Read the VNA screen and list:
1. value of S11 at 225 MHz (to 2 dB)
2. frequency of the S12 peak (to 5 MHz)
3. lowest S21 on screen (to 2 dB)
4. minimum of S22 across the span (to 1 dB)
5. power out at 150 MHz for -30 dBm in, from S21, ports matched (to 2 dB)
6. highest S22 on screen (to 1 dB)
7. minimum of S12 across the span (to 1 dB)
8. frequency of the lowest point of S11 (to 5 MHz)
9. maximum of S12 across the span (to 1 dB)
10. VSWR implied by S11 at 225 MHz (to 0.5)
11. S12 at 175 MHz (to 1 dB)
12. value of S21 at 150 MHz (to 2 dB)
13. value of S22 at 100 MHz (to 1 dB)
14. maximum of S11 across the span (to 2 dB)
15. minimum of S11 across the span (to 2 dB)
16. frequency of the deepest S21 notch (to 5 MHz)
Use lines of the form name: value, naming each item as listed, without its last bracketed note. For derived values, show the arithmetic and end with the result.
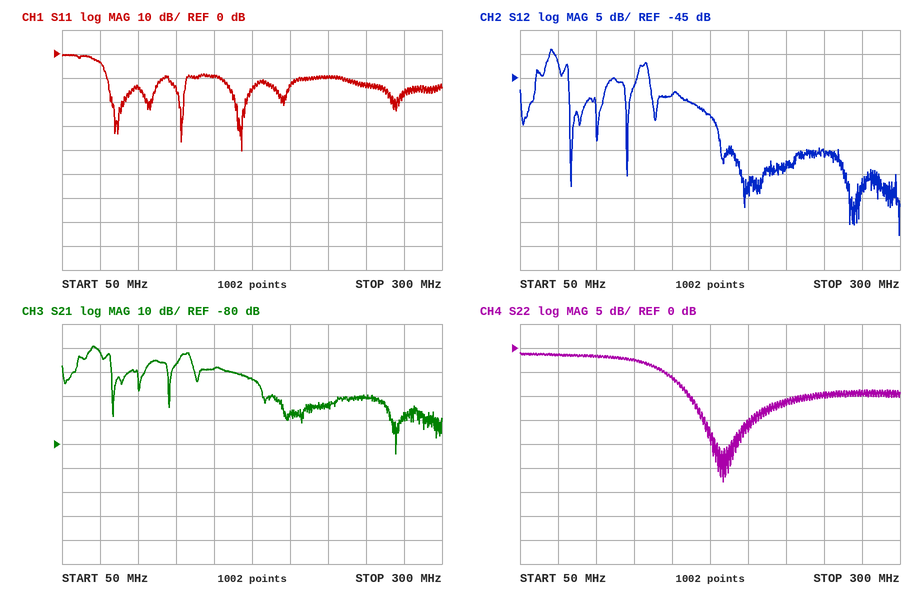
value of S11 at 225 MHz: -10 dB
frequency of the S12 peak: 70 MHz
lowest S21 on screen: -84 dB
minimum of S22 across the span: -28 dB
power out at 150 MHz for -30 dBm in, from S21, ports matched: -30 dBm + (-48 dB) = -78 dBm
highest S22 on screen: -1 dB
minimum of S12 across the span: -78 dB
frequency of the lowest point of S11: 170 MHz
maximum of S12 across the span: -39 dB
VSWR implied by S11 at 225 MHz: |Γ| = 10^(-10/20) = 0.3162; VSWR = (1 + 0.3162)/(1 − 0.3162) ≈ 1.92, so 2.0 to the nearest 0.5
S12 at 175 MHz: -53 dB
value of S21 at 150 MHz: -48 dB
value of S22 at 100 MHz: -2 dB
maximum of S11 across the span: 0 dB
minimum of S11 across the span: -40 dB
frequency of the deepest S21 notch: 270 MHz
